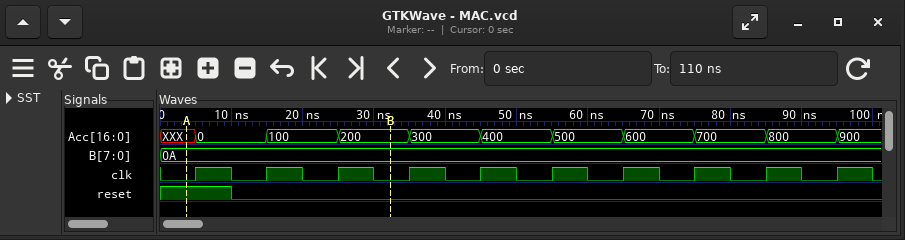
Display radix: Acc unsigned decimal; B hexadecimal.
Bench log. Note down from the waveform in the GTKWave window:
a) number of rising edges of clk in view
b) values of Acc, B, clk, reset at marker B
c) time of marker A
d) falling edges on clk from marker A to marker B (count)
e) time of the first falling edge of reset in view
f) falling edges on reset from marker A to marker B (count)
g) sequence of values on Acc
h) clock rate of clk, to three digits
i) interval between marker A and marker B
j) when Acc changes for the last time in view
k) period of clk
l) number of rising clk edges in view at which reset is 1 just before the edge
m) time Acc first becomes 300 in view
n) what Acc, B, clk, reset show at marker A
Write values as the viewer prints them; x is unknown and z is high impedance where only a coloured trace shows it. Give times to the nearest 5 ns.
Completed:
10
Acc=200, B=0A, clk=0, reset=0
5 ns
3
10 ns
1
XXX, 0, 100, 200, 300, 400, 500, 600, 700, 800, 900
100 MHz
30 ns
95 ns
10 ns
1
35 ns
Acc=XXX, B=0A, clk=0, reset=1
